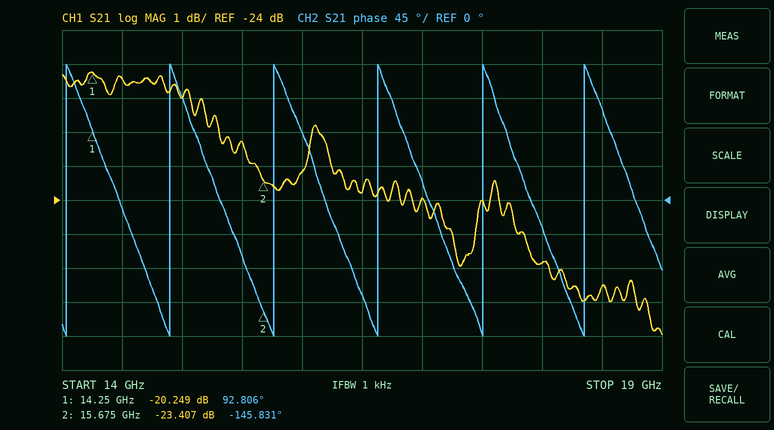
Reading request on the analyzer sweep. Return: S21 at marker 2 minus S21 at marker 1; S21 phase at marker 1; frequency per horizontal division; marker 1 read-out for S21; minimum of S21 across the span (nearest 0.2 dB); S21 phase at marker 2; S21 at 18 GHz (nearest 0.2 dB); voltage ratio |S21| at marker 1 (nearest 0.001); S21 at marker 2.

-3.158 dB
92.806°
500 MHz
-20.249 dB
-28.0 dB
-145.831°
-25.8 dB
0.097
-23.407 dB
